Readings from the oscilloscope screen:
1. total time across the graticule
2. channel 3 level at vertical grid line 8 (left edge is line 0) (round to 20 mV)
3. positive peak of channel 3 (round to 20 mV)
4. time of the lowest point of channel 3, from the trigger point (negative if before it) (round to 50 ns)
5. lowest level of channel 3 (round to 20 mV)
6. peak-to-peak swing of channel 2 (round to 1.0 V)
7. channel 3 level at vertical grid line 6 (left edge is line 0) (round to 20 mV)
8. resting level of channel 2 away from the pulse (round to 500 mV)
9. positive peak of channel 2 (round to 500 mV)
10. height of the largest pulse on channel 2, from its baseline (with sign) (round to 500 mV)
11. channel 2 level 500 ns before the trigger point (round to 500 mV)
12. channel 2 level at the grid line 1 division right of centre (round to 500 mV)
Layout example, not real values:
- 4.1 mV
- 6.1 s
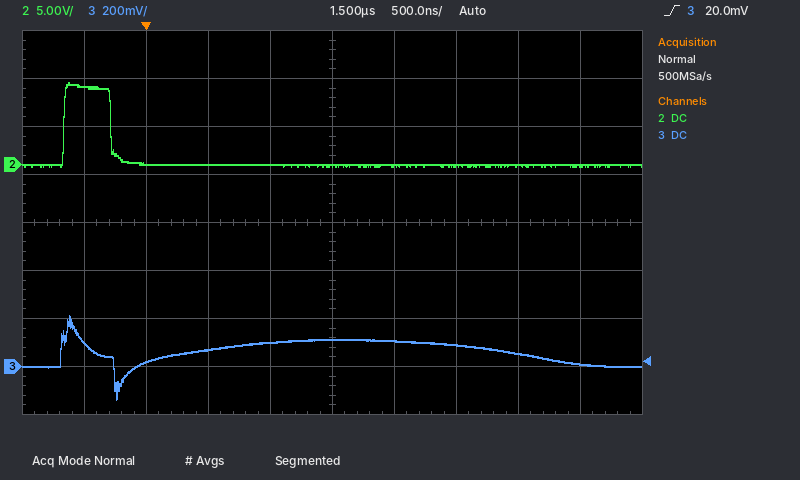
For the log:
- 5 µs
- 60 mV
- 220 mV
- -250 ns
- -140 mV
- 9.0 V
- 100 mV
- 0.0 V
- 8.5 V
- +8.5 V
- 8.0 V
- 0.0 V
